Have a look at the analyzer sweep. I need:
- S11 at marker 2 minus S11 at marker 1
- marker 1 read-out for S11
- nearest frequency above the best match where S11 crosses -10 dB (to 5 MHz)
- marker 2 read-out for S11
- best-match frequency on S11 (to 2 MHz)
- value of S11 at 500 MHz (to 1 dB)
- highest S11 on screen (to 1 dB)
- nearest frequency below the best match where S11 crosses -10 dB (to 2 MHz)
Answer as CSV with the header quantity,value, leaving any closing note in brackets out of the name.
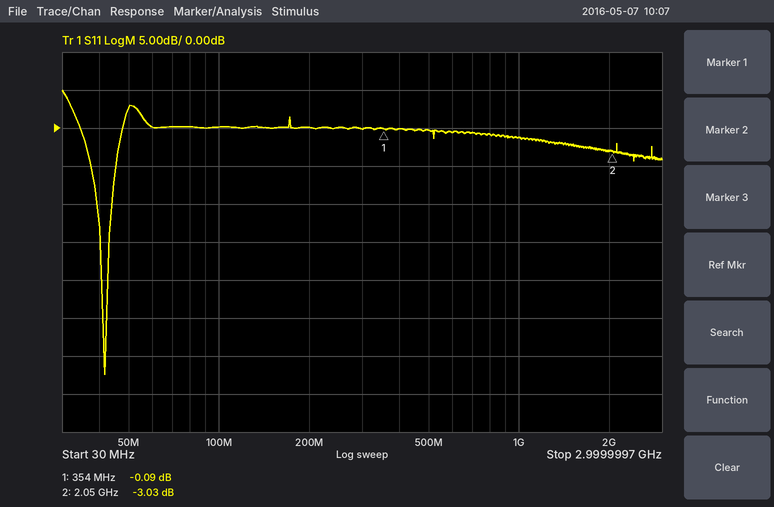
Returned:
quantity,value
S11 at marker 2 minus S11 at marker 1,-2.94 dB
marker 1 read-out for S11,-0.09 dB
nearest frequency above the best match where S11 crosses -10 dB,45 MHz
marker 2 read-out for S11,-3.03 dB
best-match frequency on S11,42 MHz
value of S11 at 500 MHz,0 dB
highest S11 on screen,5 dB
nearest frequency below the best match where S11 crosses -10 dB,40 MHz
